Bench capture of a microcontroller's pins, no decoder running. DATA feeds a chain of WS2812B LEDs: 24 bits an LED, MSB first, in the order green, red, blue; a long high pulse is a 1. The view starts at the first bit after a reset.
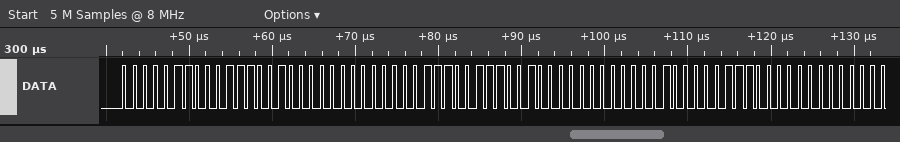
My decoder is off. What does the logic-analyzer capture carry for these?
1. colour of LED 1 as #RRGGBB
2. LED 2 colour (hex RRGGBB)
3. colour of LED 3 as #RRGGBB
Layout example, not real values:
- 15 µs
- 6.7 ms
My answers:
- #390600
- #390700
- #380800
